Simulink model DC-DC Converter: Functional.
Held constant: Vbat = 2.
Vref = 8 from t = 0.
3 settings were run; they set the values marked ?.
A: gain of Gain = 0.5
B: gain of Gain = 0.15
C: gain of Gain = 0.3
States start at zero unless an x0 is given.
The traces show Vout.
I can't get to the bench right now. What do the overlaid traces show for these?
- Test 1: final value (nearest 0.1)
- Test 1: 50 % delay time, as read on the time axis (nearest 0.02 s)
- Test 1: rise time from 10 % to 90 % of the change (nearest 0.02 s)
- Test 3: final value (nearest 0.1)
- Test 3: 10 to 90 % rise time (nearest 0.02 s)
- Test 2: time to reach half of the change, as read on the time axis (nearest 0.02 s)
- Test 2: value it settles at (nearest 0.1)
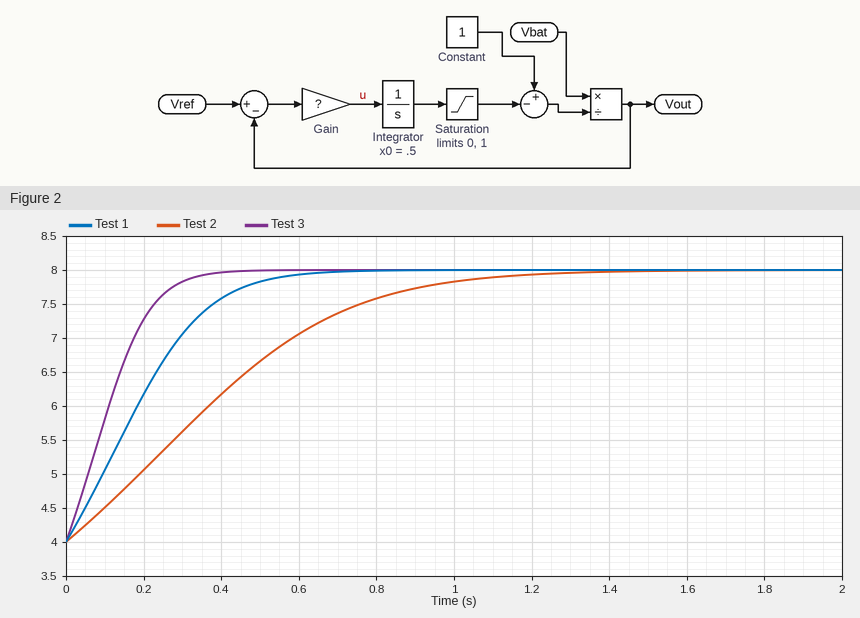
8.0
0.18 s
0.36 s
8.0
0.22 s
0.36 s
8.0
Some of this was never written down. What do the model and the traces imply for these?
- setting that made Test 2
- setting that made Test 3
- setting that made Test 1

B
A
C
